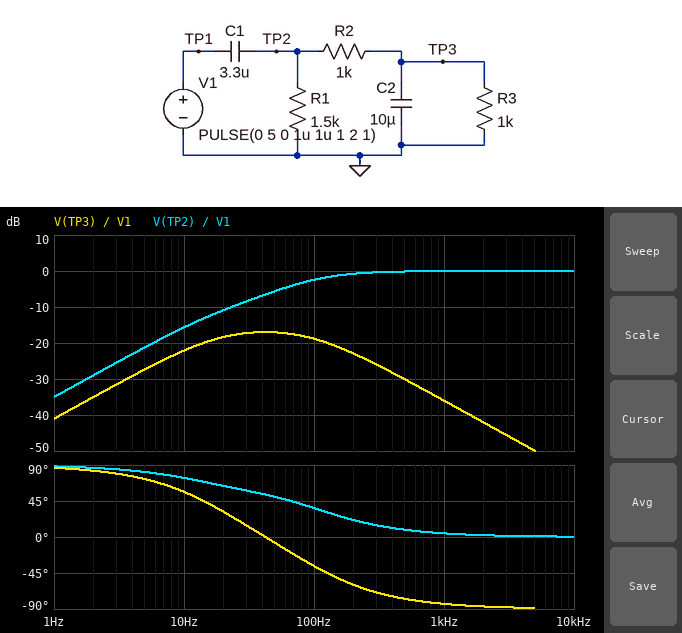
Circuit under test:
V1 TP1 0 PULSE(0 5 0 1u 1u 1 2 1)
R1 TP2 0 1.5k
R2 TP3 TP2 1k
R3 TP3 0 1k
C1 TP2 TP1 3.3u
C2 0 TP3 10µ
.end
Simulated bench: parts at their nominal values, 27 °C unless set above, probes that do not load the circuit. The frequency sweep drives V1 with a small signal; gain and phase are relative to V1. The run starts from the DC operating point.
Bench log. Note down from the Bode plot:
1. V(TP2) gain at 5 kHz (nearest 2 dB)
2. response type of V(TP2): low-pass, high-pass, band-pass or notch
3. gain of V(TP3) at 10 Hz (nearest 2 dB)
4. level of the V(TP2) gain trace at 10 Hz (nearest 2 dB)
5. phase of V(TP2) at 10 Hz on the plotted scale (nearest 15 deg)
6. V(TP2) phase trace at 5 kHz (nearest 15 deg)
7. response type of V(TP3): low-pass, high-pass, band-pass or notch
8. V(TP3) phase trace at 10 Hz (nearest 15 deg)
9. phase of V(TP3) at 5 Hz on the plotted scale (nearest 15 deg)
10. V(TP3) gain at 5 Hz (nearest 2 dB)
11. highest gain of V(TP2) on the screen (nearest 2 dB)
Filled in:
0 dB
high-pass
-22 dB
-16 dB
75 deg
0 deg
band-pass
60 deg
75 deg
-28 dB
0 dB
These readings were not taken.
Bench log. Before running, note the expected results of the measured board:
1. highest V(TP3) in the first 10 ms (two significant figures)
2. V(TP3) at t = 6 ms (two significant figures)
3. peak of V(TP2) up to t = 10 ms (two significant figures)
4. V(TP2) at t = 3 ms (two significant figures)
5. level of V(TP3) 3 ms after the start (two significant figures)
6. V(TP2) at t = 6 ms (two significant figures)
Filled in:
570 mV
490 mV
5.0 V
1.3 V
560 mV
540 mV
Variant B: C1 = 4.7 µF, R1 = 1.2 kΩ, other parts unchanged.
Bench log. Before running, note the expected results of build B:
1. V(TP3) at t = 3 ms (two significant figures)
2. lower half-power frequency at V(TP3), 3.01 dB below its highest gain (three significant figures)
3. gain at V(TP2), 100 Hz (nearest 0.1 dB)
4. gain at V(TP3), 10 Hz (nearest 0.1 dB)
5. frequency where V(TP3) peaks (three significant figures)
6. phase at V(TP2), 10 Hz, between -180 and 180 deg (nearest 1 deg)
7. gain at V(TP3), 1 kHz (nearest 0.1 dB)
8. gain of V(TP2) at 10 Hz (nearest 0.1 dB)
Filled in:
650 mV
13.4 Hz
-1.7 dB
-20.2 dB
37.9 Hz
72 deg
-36.0 dB
-13.8 dB
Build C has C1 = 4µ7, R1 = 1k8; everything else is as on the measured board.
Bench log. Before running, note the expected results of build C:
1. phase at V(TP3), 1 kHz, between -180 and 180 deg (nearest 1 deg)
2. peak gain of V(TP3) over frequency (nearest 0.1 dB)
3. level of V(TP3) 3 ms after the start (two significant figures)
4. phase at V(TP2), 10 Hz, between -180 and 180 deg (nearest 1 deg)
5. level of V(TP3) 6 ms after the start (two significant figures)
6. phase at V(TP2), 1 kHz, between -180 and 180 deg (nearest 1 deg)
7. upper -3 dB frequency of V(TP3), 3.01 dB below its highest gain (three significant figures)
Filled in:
-85 deg
-14.5 dB
700 mV
68 deg
710 mV
3 deg
96.3 Hz
